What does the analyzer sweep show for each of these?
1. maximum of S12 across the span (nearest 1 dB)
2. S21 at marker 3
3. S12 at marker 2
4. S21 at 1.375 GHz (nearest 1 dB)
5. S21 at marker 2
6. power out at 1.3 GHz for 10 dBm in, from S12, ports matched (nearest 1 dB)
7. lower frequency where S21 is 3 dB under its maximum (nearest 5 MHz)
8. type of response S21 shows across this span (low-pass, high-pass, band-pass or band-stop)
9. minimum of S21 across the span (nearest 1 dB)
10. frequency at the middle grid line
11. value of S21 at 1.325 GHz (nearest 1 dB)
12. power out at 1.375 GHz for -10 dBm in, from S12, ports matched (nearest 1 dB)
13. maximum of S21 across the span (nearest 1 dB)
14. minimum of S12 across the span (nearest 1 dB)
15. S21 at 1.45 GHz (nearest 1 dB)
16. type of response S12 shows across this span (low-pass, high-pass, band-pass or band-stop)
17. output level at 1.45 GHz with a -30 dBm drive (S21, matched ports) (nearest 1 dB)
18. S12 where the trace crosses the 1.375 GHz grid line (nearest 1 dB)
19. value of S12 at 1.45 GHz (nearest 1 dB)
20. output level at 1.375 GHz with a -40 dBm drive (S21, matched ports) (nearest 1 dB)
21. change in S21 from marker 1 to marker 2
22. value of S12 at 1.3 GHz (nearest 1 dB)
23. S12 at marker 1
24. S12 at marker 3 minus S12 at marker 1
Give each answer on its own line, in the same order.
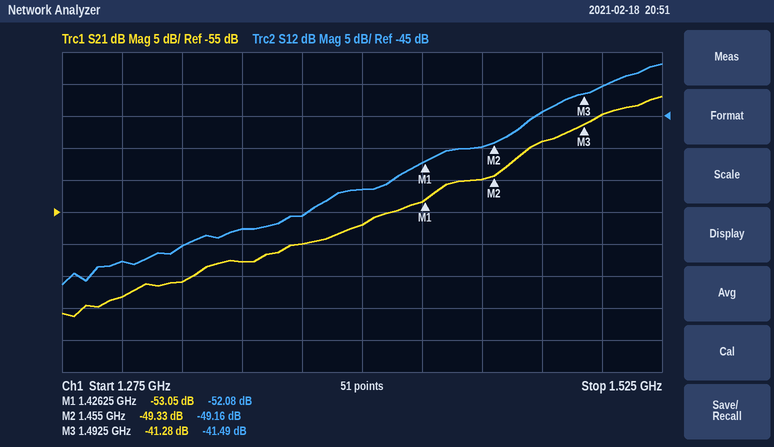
-37 dB
-41.28 dB
-49.16 dB
-60 dB
-49.33 dB
-58 dBm
1.500 GHz
high-pass
-71 dB
1.4 GHz
-66 dB
-71 dBm
-37 dB
-71 dB
-50 dB
high-pass
-80 dBm
-61 dB
-50 dB
-100 dBm
3.72 dB
-68 dB
-52.08 dB
10.59 dB
